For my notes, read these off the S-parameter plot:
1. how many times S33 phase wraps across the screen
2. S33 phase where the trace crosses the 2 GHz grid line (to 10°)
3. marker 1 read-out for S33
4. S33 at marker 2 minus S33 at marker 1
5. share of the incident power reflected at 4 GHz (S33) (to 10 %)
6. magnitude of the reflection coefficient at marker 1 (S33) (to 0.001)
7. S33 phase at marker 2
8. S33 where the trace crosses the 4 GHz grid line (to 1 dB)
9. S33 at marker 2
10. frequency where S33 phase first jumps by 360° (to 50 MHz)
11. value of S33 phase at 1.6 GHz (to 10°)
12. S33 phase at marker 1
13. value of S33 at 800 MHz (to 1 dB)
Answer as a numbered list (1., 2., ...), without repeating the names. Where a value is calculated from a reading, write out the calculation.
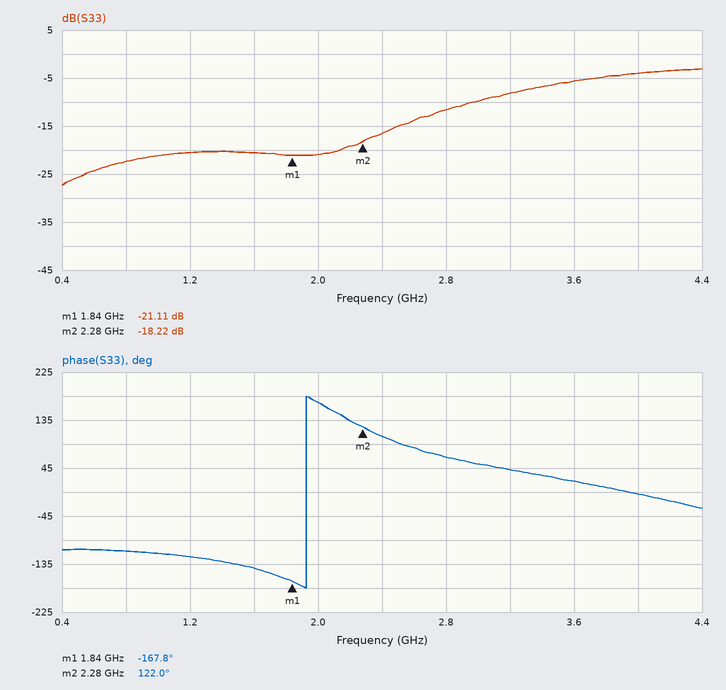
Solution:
1. 1
2. 170°
3. -21.11 dB
4. -18.22 − (-21.11) = 2.89 dB
5. 10^(-4/10) ≈ 40 %
6. 10^(-21.11/20) ≈ 0.088
7. 122.0°
8. -4 dB
9. -18.22 dB
10. 1.95 GHz
11. -140°
12. -167.8°
13. -22 dB
